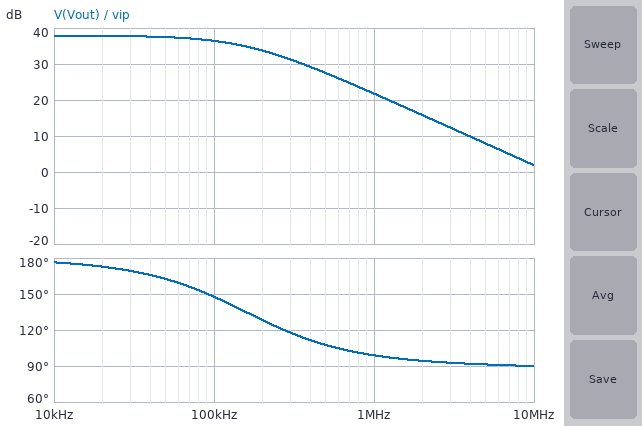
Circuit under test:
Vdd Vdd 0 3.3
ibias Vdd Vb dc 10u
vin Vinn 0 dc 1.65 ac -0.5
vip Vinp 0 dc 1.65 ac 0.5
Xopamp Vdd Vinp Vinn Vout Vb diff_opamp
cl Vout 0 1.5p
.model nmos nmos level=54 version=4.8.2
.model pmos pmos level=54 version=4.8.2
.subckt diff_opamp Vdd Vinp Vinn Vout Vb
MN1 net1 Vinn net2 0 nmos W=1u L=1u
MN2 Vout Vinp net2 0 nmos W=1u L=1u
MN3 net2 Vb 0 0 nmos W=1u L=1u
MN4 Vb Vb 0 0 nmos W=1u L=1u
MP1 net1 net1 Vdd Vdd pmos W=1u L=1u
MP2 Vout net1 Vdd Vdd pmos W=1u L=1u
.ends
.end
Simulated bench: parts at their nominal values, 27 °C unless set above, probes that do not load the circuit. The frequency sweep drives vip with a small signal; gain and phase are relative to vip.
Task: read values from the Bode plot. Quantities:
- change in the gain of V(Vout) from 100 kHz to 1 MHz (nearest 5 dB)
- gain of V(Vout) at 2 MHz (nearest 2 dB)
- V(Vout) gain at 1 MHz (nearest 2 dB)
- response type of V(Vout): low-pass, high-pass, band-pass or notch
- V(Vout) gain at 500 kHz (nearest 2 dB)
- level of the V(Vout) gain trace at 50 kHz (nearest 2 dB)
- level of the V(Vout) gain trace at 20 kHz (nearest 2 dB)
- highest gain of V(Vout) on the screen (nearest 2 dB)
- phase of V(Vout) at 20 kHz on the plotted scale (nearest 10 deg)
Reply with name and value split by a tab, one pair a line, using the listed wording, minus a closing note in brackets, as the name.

change in the gain of V(Vout) from 100 kHz to 1 MHz	-15 dB
gain of V(Vout) at 2 MHz	16 dB
V(Vout) gain at 1 MHz	22 dB
response type of V(Vout): low-pass, high-pass, band-pass or notch	low-pass
V(Vout) gain at 500 kHz	28 dB
level of the V(Vout) gain trace at 50 kHz	38 dB
level of the V(Vout) gain trace at 20 kHz	38 dB
highest gain of V(Vout) on the screen	38 dB
phase of V(Vout) at 20 kHz on the plotted scale	170 deg
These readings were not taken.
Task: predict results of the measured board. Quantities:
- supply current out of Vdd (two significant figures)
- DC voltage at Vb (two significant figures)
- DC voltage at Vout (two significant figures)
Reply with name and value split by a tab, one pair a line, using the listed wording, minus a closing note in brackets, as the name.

supply current out of Vdd	21 µA
DC voltage at Vb	430 mV
DC voltage at Vout	2.8 V
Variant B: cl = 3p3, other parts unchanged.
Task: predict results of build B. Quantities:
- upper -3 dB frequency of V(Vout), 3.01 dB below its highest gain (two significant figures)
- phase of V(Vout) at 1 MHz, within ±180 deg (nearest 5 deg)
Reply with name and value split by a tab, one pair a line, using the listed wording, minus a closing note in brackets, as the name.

upper -3 dB frequency of V(Vout), 3.01 dB below its highest gain	72 kHz
phase of V(Vout) at 1 MHz, within ±180 deg	95 deg
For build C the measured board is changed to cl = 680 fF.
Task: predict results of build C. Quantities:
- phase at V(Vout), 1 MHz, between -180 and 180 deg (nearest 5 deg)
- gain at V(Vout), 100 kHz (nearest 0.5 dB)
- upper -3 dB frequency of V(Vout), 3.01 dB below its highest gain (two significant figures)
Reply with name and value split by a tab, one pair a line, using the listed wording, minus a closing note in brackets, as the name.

phase at V(Vout), 1 MHz, between -180 and 180 deg	110 deg
gain at V(Vout), 100 kHz	37.5 dB
upper -3 dB frequency of V(Vout), 3.01 dB below its highest gain	350 kHz
